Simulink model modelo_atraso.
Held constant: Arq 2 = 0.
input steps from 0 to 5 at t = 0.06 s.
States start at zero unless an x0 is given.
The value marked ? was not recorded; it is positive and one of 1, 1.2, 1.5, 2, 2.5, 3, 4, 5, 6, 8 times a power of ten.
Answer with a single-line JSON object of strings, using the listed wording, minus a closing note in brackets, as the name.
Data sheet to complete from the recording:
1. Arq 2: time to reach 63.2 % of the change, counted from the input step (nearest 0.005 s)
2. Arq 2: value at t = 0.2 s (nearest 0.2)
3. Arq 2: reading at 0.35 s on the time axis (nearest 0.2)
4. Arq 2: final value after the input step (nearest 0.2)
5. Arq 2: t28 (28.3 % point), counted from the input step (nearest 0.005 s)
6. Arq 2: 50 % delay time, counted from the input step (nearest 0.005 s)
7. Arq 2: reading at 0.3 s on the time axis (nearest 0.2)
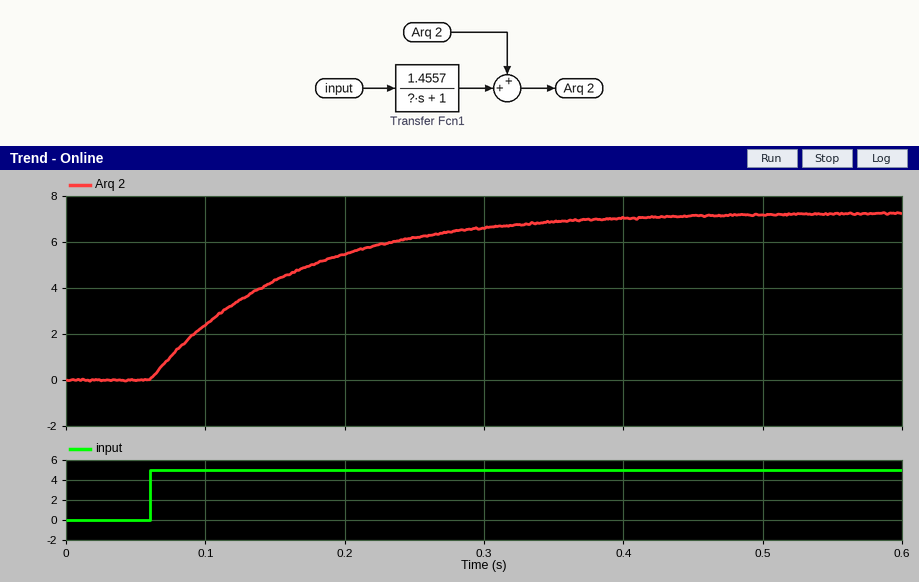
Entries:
{"Arq 2: time to reach 63.2 % of the change, counted from the input step": "0.100 s", "Arq 2: value at t = 0.2 s": "5.4", "Arq 2: reading at 0.35 s on the time axis": "6.8", "Arq 2: final value after the input step": "7.2", "Arq 2: t28 (28.3 % point), counted from the input step": "0.035 s", "Arq 2: 50 % delay time, counted from the input step": "0.070 s", "Arq 2: reading at 0.3 s on the time axis": "6.6"}
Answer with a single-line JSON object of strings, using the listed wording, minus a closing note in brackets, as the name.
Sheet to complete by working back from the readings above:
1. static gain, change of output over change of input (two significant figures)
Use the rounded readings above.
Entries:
{"static gain, change of output over change of input": "1.4"}
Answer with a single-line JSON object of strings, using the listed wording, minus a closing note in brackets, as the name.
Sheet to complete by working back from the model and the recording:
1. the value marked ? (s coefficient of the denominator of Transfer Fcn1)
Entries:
{"the value marked ?": "0.1"}
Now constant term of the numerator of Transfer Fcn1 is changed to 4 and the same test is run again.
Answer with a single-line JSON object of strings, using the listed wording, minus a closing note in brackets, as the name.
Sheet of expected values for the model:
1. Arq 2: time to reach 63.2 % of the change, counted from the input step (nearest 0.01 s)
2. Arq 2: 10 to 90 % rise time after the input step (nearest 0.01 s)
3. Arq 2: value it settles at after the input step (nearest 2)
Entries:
{"Arq 2: time to reach 63.2 % of the change, counted from the input step": "0.10 s", "Arq 2: 10 to 90 % rise time after the input step": "0.22 s", "Arq 2: value it settles at after the input step": "20"}
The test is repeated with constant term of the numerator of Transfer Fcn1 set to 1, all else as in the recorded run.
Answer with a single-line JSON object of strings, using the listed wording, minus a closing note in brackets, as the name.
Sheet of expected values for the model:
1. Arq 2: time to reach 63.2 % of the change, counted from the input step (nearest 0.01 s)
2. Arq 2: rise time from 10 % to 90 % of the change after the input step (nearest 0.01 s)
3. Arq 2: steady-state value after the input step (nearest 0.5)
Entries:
{"Arq 2: time to reach 63.2 % of the change, counted from the input step": "0.10 s", "Arq 2: rise time from 10 % to 90 % of the change after the input step": "0.22 s", "Arq 2: steady-state value after the input step": "5.0"}
